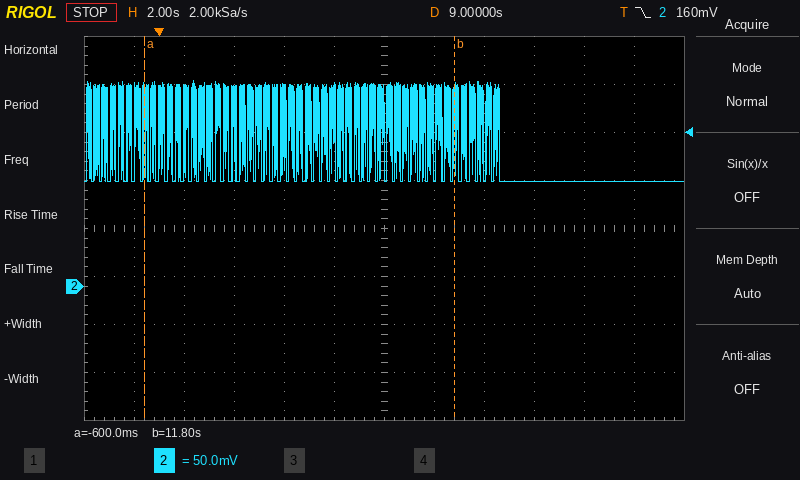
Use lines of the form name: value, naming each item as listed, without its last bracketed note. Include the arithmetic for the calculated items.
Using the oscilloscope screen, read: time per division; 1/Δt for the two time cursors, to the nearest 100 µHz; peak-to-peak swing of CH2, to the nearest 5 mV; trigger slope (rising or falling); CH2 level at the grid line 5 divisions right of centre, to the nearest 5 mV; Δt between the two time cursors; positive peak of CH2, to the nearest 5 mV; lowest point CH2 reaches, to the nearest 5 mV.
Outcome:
time per division: 2 s
1/Δt for the two time cursors, to the nearest 100 µHz: 1 / 12.4 s ≈ 80.6 mHz
peak-to-peak swing of CH2, to the nearest 5 mV: 215 mV − (110 mV) = 105 mV
trigger slope: falling
CH2 level at the grid line 5 divisions right of centre, to the nearest 5 mV: 110 mV
Δt between the two time cursors: 11.8 s − (-600 ms) = 12.4 s
positive peak of CH2, to the nearest 5 mV: 215 mV
lowest point CH2 reaches, to the nearest 5 mV: 110 mV
